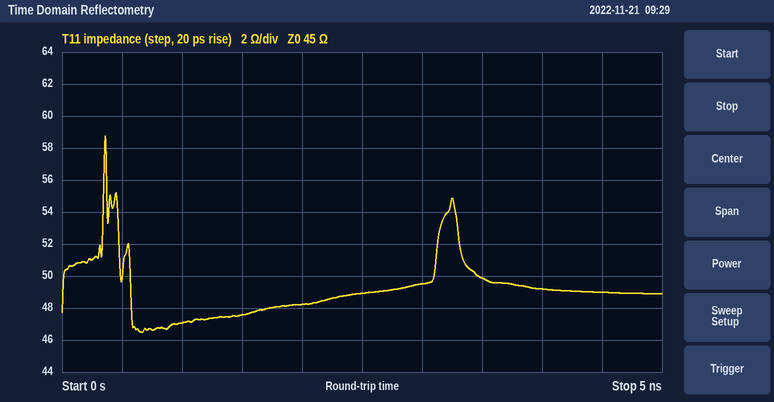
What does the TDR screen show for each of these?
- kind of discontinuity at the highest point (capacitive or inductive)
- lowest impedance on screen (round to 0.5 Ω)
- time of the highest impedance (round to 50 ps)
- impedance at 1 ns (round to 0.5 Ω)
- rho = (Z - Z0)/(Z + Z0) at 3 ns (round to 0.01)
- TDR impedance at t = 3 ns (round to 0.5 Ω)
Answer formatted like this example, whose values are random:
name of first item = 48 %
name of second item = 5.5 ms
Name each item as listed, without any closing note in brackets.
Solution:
kind of discontinuity at the highest point = inductive
lowest impedance on screen = 46.5 Ω
time of the highest impedance = 350 ps
impedance at 1 ns = 47.0 Ω
rho = (Z - Z0)/(Z + Z0) at 3 ns = +0.05
TDR impedance at t = 3 ns = 49.5 Ω
